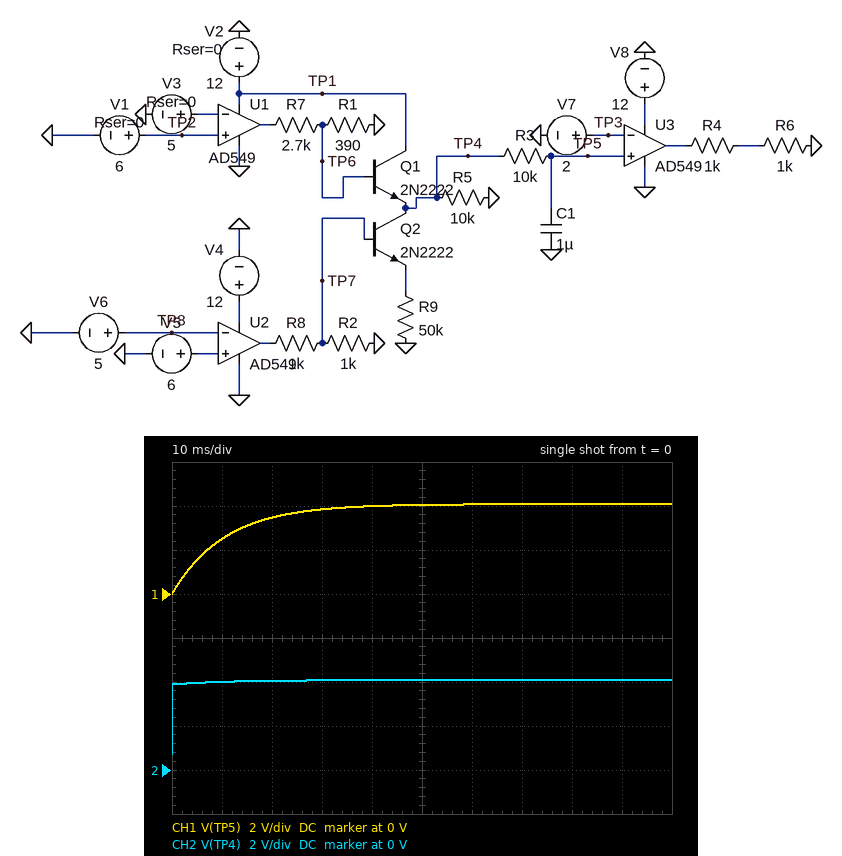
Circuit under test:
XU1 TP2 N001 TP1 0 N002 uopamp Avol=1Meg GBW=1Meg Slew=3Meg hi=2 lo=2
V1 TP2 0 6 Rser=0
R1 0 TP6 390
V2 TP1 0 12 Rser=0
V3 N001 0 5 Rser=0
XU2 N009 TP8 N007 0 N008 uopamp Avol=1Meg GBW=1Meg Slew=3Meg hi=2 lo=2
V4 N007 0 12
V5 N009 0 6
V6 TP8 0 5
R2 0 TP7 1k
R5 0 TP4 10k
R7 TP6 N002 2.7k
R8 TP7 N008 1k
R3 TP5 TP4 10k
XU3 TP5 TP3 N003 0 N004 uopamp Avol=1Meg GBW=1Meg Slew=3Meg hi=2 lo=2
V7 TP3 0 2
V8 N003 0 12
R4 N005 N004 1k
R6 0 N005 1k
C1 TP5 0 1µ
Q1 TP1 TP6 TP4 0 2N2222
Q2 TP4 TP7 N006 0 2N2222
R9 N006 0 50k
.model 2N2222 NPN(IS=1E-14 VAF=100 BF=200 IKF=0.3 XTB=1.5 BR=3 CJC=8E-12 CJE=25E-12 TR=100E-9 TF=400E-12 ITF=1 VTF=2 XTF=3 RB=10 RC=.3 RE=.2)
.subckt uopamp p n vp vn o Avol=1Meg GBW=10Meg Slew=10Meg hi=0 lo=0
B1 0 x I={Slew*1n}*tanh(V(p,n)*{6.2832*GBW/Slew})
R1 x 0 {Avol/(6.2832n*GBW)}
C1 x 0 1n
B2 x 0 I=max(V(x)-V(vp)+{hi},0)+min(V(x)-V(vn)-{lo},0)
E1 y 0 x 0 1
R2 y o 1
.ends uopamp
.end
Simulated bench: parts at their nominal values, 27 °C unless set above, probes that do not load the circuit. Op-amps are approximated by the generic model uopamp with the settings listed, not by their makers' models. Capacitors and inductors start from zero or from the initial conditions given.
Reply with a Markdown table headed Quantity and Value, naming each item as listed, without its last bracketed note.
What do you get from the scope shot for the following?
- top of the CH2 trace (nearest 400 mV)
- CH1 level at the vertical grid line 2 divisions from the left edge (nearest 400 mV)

| Quantity | Value |
|---|---|
| top of the CH2 trace | 4.0 V |
| CH1 level at the vertical grid line 2 divisions from the left edge | 3.6 V |
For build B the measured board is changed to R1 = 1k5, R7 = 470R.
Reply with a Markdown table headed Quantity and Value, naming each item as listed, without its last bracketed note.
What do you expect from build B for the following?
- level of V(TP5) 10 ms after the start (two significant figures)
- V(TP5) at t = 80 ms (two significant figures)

| Quantity | Value |
|---|---|
| level of V(TP5) 10 ms after the start | 4.4 V |
| V(TP5) at t = 80 ms | 7.0 V |
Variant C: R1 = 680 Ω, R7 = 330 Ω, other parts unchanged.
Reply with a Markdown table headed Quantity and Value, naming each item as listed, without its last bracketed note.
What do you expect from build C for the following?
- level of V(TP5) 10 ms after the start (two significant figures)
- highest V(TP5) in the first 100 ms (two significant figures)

| Quantity | Value |
|---|---|
| level of V(TP5) 10 ms after the start | 3.8 V |
| highest V(TP5) in the first 100 ms | 6.1 V |
